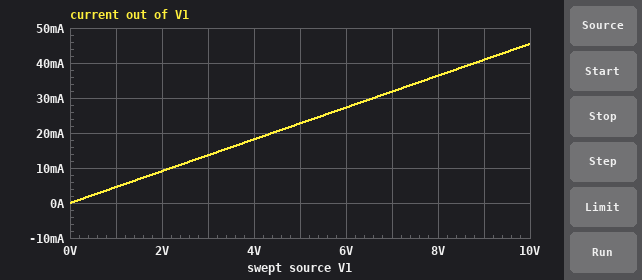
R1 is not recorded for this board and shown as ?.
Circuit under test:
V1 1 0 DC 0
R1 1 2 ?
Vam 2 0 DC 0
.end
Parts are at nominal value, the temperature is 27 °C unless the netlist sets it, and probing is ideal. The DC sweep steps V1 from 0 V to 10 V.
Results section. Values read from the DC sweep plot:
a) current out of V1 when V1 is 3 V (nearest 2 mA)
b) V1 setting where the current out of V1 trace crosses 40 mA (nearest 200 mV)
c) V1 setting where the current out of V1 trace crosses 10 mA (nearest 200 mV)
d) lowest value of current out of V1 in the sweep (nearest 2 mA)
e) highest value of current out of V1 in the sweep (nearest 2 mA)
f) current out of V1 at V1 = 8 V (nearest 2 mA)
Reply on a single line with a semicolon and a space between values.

14 mA; 8.8 V; 2.2 V; 0 A; 46 mA; 36 mA
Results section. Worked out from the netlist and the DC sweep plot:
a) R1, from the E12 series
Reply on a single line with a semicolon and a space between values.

220 Ω
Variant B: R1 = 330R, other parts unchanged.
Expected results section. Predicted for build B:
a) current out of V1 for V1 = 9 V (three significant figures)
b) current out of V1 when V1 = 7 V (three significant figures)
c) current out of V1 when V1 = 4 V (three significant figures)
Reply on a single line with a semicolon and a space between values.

27.3 mA; 21.2 mA; 12.1 mA
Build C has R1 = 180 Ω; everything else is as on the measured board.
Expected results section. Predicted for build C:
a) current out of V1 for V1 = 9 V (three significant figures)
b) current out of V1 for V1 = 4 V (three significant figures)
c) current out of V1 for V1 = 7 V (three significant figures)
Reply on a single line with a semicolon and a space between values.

50.0 mA; 22.2 mA; 38.9 mA
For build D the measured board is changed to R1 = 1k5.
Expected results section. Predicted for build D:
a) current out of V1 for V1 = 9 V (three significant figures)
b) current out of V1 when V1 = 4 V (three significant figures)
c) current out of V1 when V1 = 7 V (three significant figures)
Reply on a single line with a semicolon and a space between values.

6.00 mA; 2.67 mA; 4.67 mA
